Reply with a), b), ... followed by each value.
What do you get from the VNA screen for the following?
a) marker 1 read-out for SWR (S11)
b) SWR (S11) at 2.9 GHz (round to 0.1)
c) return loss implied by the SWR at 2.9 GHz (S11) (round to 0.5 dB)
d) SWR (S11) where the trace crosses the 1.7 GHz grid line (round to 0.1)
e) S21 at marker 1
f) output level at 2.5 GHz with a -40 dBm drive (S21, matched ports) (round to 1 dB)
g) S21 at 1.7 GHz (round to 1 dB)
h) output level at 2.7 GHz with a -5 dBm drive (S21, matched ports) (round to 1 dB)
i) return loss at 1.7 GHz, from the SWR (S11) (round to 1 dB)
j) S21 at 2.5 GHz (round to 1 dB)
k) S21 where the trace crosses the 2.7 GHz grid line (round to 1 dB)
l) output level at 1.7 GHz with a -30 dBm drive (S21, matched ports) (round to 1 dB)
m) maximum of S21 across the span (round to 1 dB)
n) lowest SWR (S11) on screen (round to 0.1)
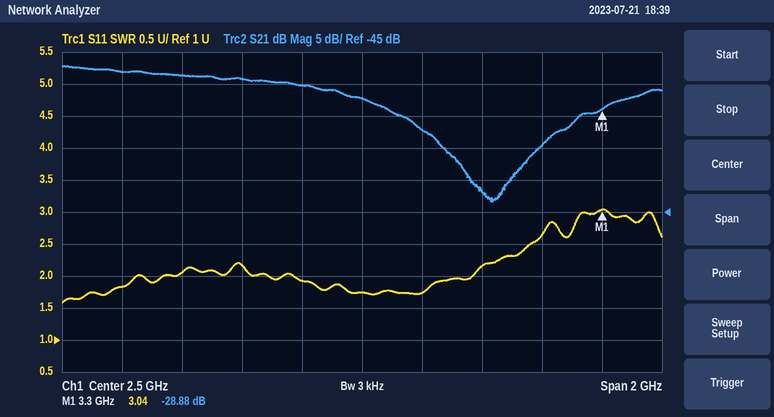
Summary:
a) 3.04
b) 2.2
c) 8.5 dB
d) 1.8
e) -28.88 dB
f) -67 dBm
g) -23 dB
h) -37 dBm
i) 11 dB
j) -27 dB
k) -32 dB
l) -53 dBm
m) -22 dB
n) 1.6
